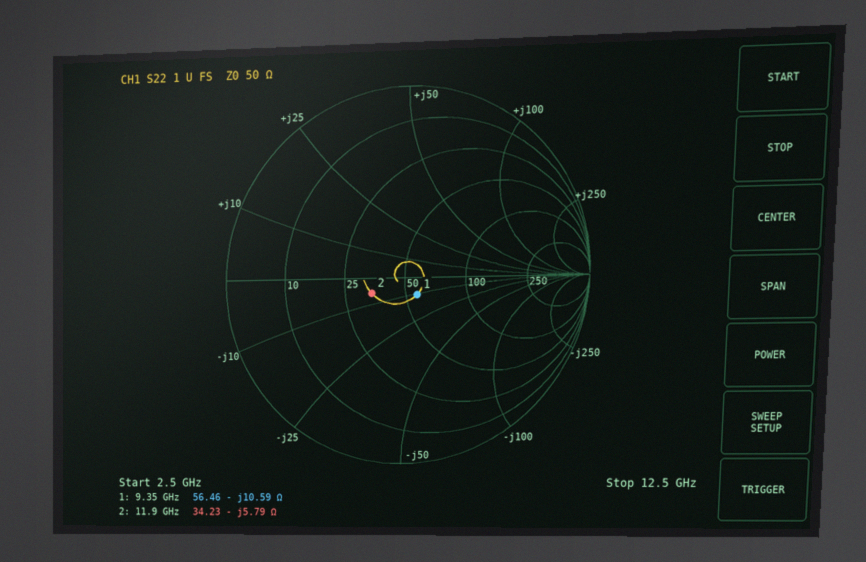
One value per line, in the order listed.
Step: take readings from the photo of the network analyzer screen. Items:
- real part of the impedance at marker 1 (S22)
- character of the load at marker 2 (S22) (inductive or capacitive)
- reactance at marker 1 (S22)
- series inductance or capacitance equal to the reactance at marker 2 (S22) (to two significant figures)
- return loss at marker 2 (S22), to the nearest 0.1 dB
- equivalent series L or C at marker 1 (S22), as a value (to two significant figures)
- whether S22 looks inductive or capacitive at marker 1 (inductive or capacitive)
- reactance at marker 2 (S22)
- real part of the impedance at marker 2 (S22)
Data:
56.46 Ω
capacitive
-10.59 Ω
2.3 pF
14.0 dB
1.6 pF
capacitive
-5.79 Ω
34.23 Ω
